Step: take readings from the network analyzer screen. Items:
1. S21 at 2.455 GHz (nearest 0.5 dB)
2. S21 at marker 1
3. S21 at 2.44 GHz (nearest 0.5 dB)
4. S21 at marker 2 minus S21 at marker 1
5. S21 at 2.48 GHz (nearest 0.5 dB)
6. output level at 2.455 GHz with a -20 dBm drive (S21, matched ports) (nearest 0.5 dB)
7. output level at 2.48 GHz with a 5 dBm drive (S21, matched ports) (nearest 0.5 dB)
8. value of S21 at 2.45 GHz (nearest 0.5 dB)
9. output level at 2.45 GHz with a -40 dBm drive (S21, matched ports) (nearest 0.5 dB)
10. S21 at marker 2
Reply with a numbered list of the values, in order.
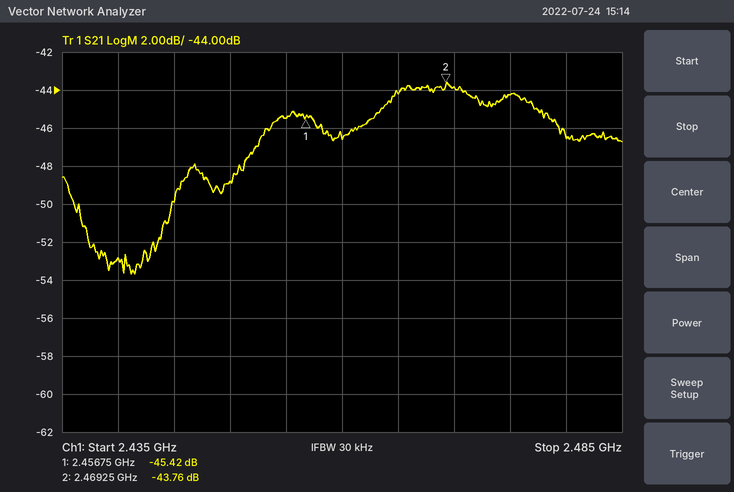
1. -45.5 dB
2. -45.42 dB
3. -53.0 dB
4. 1.66 dB
5. -46.5 dB
6. -65.5 dBm
7. -41.5 dBm
8. -49.0 dB
9. -89.0 dBm
10. -43.76 dB
